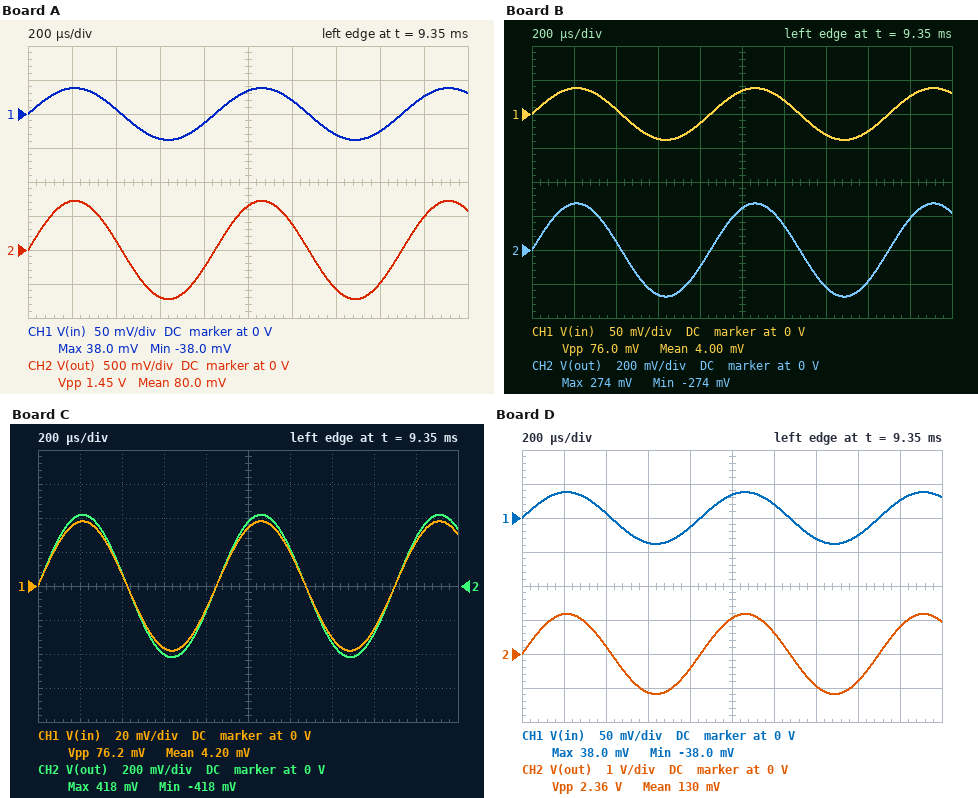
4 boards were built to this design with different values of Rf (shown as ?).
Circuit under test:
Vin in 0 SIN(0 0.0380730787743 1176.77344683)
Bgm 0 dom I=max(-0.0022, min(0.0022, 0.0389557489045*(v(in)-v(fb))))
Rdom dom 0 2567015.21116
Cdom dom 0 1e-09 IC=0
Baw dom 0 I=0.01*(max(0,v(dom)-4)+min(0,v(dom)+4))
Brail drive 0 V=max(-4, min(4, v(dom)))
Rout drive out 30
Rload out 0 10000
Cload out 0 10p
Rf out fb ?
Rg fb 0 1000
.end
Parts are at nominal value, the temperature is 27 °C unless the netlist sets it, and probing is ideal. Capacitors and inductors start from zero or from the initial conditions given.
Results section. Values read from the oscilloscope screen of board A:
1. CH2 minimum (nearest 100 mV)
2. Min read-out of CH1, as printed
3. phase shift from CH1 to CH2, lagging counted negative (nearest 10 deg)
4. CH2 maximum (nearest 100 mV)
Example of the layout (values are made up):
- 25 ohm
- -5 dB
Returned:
- -700 mV
- -38.0 mV
- 0 deg
- 700 mV
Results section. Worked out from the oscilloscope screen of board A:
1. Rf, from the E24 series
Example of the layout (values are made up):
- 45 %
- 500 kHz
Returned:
- 18 kΩ
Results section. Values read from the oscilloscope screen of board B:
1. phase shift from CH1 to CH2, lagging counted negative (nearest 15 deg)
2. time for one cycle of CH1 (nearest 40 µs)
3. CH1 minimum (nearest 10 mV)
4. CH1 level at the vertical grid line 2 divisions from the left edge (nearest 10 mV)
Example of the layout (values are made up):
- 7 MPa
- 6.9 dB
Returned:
- 0 deg
- 840 µs
- -40 mV
- 10 mV
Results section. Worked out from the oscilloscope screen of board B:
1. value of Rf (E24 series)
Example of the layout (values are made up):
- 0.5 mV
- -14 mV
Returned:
- 6.2 kΩ
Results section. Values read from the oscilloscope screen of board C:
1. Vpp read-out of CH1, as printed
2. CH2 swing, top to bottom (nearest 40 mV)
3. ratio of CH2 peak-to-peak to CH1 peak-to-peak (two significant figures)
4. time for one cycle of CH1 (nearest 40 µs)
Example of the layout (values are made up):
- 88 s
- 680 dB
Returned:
- 76.2 mV
- 840 mV
- 11
- 840 µs
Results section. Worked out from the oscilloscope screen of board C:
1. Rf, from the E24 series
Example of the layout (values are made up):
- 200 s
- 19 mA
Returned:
- 10 kΩ
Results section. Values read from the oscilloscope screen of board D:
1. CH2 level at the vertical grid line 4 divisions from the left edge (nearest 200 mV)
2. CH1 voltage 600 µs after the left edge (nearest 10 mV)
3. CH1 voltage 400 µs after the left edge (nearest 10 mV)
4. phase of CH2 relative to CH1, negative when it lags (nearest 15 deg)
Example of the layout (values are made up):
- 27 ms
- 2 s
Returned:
- -400 mV
- -40 mV
- 10 mV
- 0 deg
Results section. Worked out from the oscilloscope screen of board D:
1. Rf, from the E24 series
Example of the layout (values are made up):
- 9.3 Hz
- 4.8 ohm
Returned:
- 30 kΩ
